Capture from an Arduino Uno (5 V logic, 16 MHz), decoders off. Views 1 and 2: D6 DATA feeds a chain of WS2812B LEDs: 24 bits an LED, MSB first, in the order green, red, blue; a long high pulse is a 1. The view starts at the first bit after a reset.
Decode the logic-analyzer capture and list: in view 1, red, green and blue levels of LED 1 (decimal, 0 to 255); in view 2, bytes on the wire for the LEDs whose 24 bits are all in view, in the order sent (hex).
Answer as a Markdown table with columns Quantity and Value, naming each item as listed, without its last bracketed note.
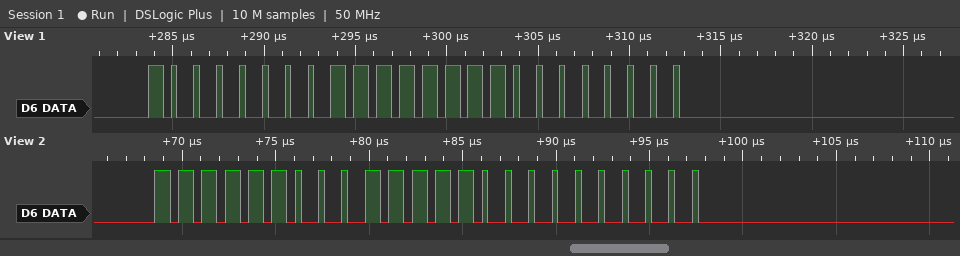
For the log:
| Quantity | Value |
|---|---|
| in view 1, red, green and blue levels of LED 1 | 255, 128, 0 |
| in view 2, bytes on the wire for the LEDs whose 24 bits are all in view, in the order sent | FC 7C 00 |
